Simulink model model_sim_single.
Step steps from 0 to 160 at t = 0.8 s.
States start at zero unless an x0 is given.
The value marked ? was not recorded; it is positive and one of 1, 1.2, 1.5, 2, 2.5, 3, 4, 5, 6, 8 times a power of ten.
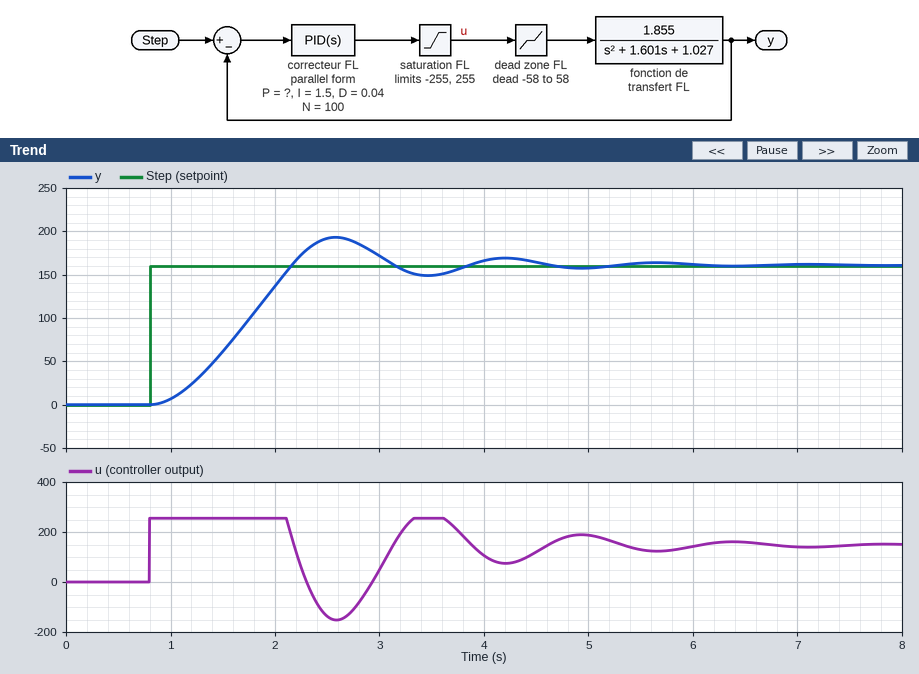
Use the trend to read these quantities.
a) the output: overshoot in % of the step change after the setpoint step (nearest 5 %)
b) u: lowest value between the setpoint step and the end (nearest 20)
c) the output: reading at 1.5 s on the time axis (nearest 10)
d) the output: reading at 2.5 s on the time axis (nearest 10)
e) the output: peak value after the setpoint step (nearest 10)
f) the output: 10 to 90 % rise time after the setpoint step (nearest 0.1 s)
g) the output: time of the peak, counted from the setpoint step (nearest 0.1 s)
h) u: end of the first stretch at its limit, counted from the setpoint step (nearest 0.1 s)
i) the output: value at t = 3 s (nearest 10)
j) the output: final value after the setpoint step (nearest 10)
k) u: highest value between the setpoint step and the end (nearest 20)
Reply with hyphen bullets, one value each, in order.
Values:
- 20 %
- -160
- 60
- 190
- 190
- 0.9 s
- 1.8 s
- 1.3 s
- 170
- 160
- 260
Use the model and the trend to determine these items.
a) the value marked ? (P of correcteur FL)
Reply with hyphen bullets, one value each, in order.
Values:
- 10
